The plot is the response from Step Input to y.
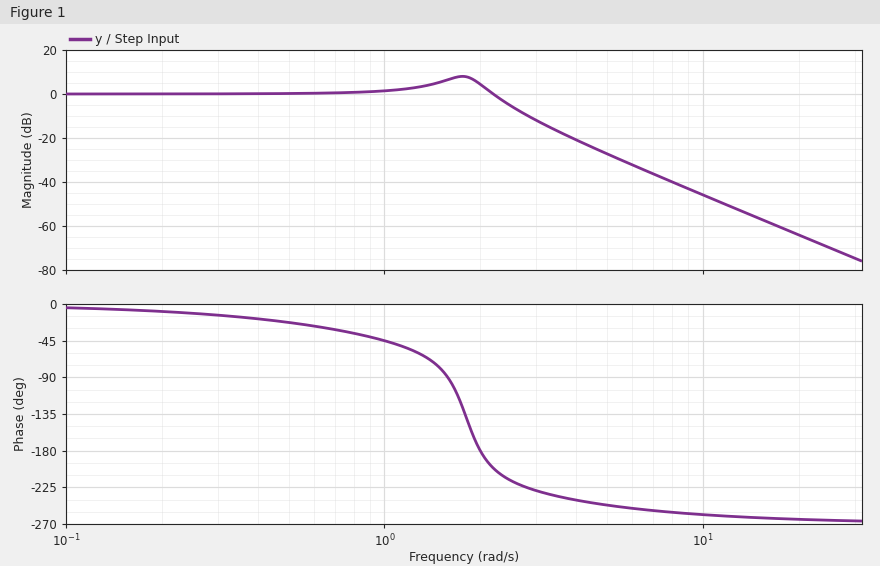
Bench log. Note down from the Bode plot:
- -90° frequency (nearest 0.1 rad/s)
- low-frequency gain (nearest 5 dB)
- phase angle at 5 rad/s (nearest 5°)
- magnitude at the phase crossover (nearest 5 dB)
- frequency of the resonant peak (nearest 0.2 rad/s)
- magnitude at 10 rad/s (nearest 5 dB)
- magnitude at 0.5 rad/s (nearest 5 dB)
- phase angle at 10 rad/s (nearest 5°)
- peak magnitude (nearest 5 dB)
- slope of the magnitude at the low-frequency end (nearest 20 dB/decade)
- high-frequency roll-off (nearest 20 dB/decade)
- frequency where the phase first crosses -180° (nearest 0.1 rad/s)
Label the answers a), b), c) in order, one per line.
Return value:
a) 1.6 rad/s
b) 0 dB
c) -245°
d) 5 dB
e) 1.8 rad/s
f) -45 dB
g) 0 dB
h) -260°
i) 10 dB
j) 0 dB/decade
k) -60 dB/decade
l) 2.0 rad/s
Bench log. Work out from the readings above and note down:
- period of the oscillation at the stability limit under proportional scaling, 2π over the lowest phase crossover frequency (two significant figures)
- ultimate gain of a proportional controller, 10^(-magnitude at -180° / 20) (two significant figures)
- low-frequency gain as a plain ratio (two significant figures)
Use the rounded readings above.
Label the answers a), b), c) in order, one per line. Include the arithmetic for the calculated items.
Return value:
a) 2π / 2 = 3.1 s
b) 10^(-5 / 20) = 0.56
c) 10^(0 / 20) = 1.0
